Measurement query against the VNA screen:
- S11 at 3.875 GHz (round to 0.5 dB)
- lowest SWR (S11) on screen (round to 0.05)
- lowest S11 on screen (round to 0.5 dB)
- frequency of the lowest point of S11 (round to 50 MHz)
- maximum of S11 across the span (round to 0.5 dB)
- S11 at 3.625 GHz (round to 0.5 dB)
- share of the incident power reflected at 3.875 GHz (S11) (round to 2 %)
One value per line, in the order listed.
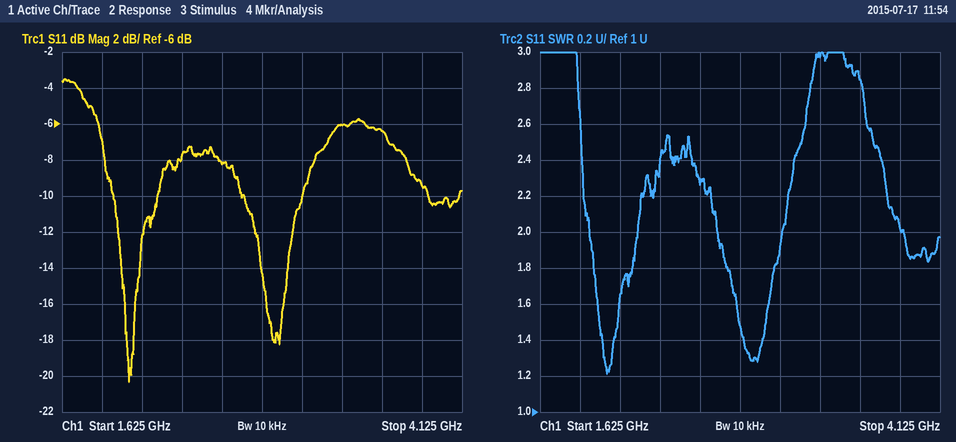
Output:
-9.5 dB
1.20
-20.5 dB
2.05 GHz
-3.5 dB
-6.5 dB
12 %
